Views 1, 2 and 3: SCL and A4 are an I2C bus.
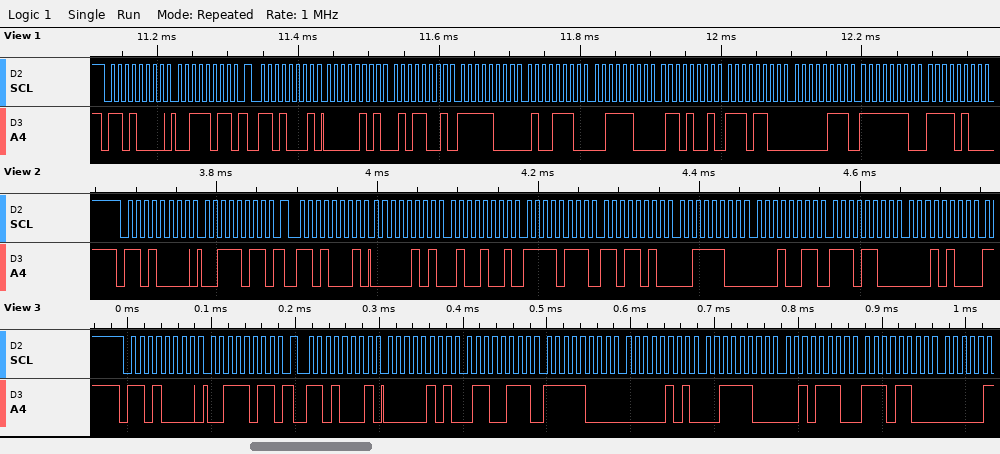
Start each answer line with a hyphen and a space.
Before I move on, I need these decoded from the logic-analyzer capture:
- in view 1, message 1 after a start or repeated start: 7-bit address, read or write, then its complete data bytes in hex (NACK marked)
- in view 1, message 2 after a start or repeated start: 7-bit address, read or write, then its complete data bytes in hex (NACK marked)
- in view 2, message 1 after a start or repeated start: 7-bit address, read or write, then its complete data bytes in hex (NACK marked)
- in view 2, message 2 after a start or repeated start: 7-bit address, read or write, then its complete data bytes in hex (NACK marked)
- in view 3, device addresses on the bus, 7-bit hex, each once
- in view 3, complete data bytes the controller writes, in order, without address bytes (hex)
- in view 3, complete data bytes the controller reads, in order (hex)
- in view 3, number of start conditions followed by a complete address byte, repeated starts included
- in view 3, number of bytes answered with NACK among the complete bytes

- 0x68 write: 3B
- 0x68 read: 05 59 F8 4E 3C 69 EC 07 FE F4
- 0x68 write: 3B
- 0x68 read: 05 49 F7 DA 3C 13 EC 14
- 0x68
- 3B
- 05 67 F8 05 3C 2E EC
- 2
- 0
